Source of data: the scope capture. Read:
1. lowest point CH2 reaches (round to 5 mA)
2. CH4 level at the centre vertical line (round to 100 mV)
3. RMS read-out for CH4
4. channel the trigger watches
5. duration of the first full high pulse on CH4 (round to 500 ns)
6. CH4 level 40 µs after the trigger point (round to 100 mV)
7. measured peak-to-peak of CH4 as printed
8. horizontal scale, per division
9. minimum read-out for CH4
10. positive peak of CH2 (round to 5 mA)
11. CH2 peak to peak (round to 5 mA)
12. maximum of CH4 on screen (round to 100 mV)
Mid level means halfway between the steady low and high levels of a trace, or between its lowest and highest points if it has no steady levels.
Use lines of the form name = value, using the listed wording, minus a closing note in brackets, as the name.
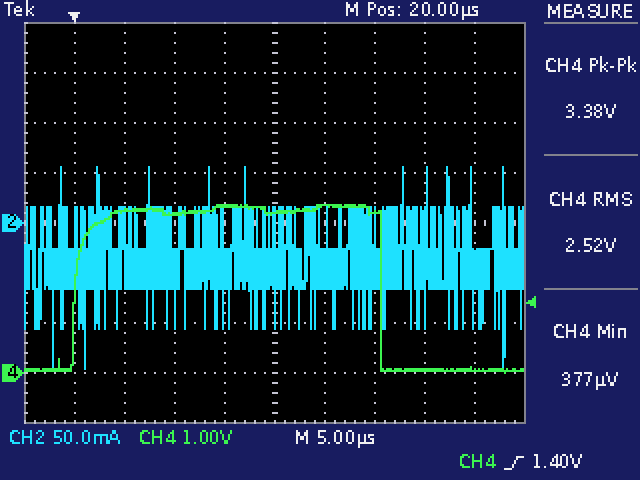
lowest point CH2 reaches = -145 mA
CH4 level at the centre vertical line = 3.2 V
RMS read-out for CH4 = 2.52 V
channel the trigger watches = CH4
duration of the first full high pulse on CH4 = 30.5 µs
CH4 level 40 µs after the trigger point = 100 mV
measured peak-to-peak of CH4 as printed = 3.38 V
horizontal scale, per division = 5 µs
minimum read-out for CH4 = 377 µV
positive peak of CH2 = 55 mA
CH2 peak to peak = 200 mA
maximum of CH4 on screen = 3.4 V
